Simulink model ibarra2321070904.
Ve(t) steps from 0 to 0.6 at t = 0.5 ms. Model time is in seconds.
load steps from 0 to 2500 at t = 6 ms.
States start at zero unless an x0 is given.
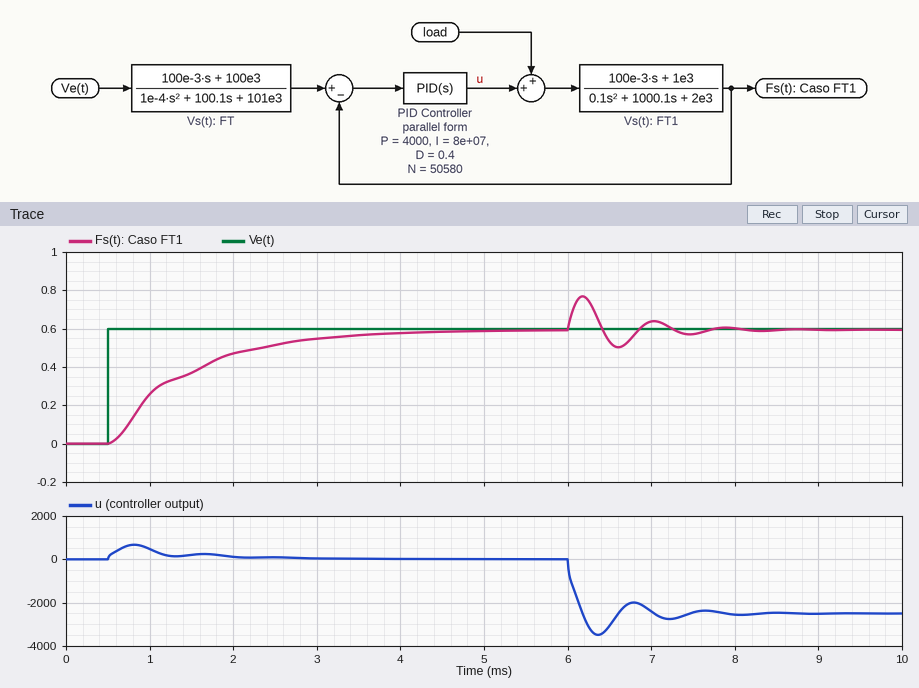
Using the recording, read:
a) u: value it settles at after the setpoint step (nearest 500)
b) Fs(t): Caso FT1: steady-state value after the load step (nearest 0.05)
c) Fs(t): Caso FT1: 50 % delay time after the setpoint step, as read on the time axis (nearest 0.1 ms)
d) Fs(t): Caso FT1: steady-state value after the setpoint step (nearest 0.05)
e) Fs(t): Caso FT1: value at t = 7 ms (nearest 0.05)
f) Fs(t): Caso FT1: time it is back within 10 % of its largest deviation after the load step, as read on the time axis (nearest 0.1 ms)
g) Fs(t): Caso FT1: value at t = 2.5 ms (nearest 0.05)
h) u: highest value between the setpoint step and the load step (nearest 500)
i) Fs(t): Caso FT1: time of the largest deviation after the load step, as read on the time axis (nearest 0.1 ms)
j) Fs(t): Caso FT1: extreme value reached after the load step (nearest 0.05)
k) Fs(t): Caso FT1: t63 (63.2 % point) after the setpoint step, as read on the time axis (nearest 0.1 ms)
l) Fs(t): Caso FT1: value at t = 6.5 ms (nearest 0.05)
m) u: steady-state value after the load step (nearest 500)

0
0.60
1.1 ms
0.60
0.65
7.6 ms
0.50
500
6.2 ms
0.75
1.5 ms
0.55
-2500
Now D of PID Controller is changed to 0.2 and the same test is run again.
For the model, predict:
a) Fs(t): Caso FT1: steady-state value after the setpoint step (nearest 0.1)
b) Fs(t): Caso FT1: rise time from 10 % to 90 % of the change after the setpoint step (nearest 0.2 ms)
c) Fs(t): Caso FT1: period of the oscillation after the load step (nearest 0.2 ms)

0.6
2.0 ms
0.8 ms
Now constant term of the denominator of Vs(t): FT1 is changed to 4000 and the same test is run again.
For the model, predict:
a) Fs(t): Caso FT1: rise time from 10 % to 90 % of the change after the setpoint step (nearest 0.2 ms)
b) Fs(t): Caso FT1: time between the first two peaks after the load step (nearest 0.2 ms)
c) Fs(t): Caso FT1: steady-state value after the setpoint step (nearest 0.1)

2.0 ms
0.8 ms
0.6
